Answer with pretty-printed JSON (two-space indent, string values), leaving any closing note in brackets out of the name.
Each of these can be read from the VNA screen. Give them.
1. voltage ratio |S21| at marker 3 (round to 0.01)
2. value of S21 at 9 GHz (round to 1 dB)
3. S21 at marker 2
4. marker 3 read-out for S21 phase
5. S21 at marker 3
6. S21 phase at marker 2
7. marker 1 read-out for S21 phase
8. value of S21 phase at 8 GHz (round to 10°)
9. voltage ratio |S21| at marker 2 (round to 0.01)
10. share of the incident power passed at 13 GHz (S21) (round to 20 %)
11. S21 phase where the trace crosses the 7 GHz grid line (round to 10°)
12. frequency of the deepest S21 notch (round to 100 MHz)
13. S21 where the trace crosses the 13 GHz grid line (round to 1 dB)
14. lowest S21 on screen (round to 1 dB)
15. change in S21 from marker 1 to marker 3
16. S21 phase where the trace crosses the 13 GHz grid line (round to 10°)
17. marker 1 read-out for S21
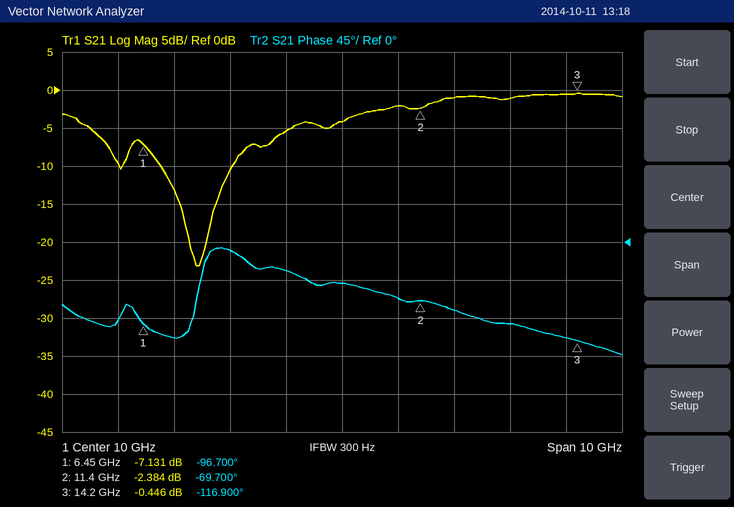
{
  "voltage ratio |S21| at marker 3": "0.95",
  "value of S21 at 9 GHz": "-5 dB",
  "S21 at marker 2": "-2.384 dB",
  "marker 3 read-out for S21 phase": "-116.900°",
  "S21 at marker 3": "-0.446 dB",
  "S21 phase at marker 2": "-69.700°",
  "marker 1 read-out for S21 phase": "-96.700°",
  "value of S21 phase at 8 GHz": "-10°",
  "voltage ratio |S21| at marker 2": "0.76",
  "share of the incident power passed at 13 GHz (S21)": "80 %",
  "S21 phase where the trace crosses the 7 GHz grid line": "-110°",
  "frequency of the deepest S21 notch": "7.4 GHz",
  "S21 where the trace crosses the 13 GHz grid line": "-1 dB",
  "lowest S21 on screen": "-23 dB",
  "change in S21 from marker 1 to marker 3": "6.685 dB",
  "S21 phase where the trace crosses the 13 GHz grid line": "-100°",
  "marker 1 read-out for S21": "-7.131 dB"
}
